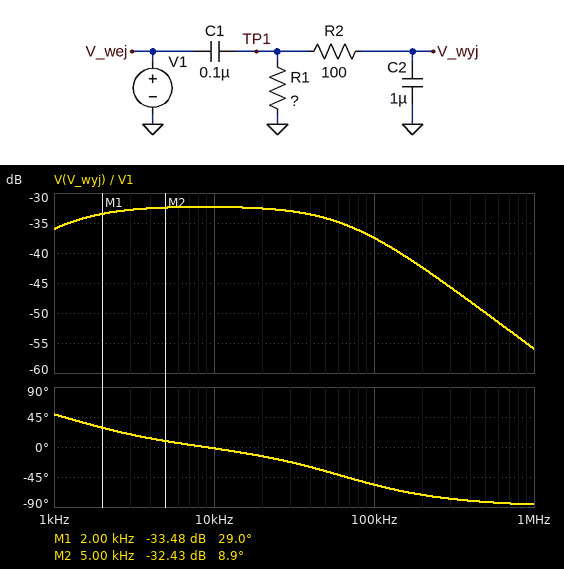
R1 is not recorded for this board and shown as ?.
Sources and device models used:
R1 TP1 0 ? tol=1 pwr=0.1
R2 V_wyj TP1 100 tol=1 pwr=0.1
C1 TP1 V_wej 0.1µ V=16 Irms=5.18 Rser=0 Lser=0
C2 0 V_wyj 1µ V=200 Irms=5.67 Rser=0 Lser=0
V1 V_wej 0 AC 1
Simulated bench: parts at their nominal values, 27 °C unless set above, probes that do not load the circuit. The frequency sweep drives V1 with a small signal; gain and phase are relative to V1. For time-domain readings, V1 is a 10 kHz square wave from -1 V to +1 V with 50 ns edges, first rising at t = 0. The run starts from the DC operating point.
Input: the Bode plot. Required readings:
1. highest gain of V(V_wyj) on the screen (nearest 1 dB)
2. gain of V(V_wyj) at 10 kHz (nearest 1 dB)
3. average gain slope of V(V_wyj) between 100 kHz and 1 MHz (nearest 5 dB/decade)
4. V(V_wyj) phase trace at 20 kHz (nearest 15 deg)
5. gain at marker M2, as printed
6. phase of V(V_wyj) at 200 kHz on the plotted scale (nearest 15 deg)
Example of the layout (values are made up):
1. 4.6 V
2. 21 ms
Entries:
1. -32 dB
2. -32 dB
3. -20 dB/decade
4. -15 deg
5. -32.43 dB
6. -75 deg
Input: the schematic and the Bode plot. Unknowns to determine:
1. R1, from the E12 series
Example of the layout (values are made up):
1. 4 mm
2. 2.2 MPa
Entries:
1. 33 Ω
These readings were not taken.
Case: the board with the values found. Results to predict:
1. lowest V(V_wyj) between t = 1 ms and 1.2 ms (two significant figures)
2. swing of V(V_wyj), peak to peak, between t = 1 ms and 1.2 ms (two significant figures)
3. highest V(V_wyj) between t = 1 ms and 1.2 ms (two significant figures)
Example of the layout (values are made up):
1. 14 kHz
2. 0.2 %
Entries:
1. -27 mV
2. 54 mV
3. 27 mV
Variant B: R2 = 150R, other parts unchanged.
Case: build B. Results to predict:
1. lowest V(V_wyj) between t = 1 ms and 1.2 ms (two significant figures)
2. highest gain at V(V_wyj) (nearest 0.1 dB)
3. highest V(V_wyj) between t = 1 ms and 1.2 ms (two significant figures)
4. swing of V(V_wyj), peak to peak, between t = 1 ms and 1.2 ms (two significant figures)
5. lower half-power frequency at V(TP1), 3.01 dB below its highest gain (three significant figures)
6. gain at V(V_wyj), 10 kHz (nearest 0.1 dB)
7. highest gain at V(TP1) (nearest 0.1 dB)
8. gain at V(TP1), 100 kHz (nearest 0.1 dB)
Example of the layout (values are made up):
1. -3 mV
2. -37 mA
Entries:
1. -19 mV
2. -35.0 dB
3. 19 mV
4. 38 mV
5. 59.0 kHz
6. -35.1 dB
7. 0 dB
8. -1.3 dB
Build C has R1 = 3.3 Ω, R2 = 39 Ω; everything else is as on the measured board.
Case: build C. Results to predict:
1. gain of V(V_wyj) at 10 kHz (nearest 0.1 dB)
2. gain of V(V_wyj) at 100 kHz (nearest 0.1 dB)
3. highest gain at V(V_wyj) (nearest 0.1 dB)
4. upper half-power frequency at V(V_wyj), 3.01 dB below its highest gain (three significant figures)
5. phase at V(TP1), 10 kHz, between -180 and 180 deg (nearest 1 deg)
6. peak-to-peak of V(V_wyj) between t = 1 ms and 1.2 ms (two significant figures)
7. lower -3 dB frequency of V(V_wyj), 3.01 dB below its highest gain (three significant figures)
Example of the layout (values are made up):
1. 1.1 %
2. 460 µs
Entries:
1. -42.7 dB
2. -42.3 dB
3. -42.2 dB
4. 531 kHz
5. 87 deg
6. 23 mV
7. 3.71 kHz
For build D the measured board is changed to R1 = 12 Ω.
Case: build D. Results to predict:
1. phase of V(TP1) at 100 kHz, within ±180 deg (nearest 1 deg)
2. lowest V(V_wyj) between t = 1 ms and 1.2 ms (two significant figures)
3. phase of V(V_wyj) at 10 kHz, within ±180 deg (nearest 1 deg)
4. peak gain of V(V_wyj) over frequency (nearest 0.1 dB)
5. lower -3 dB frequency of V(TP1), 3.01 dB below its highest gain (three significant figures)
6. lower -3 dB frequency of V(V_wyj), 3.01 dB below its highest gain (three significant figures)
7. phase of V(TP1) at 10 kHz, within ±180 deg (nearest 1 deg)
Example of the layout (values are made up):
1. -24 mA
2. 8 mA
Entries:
1. 56 deg
2. -12 mV
3. 4 deg
4. -39.5 dB
5. 149 kHz
6. 1.39 kHz
7. 85 deg
